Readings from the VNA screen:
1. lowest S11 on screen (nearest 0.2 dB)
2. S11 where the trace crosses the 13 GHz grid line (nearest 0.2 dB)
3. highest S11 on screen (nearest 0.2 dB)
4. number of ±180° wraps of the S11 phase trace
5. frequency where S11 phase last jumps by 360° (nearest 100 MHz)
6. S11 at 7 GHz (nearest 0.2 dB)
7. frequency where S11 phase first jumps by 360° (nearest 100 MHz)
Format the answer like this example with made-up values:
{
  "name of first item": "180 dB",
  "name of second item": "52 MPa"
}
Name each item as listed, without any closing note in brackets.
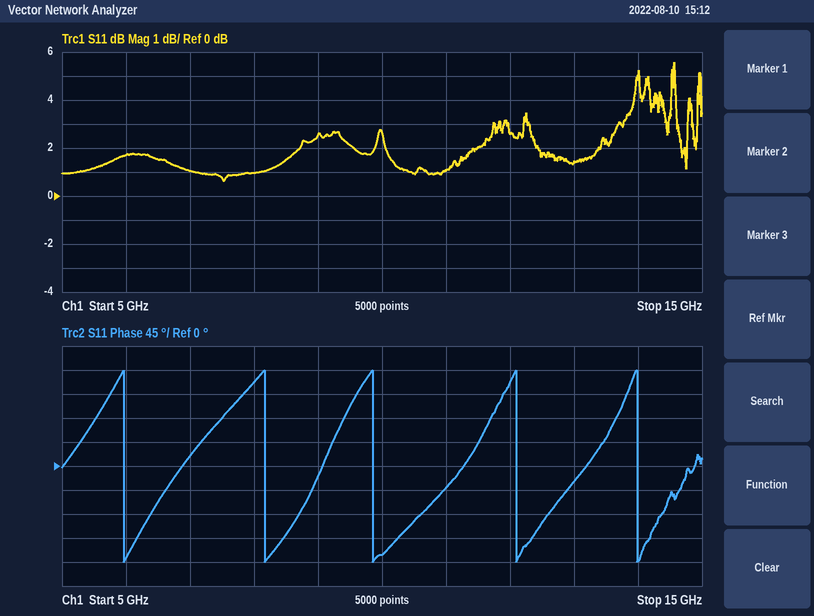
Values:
{
  "lowest S11 on screen": "0.6 dB",
  "S11 where the trace crosses the 13 GHz grid line": "1.4 dB",
  "highest S11 on screen": "5.6 dB",
  "number of ±180° wraps of the S11 phase trace": "5",
  "frequency where S11 phase last jumps by 360°": "14.0 GHz",
  "S11 at 7 GHz": "1.0 dB",
  "frequency where S11 phase first jumps by 360°": "6.0 GHz"
}
